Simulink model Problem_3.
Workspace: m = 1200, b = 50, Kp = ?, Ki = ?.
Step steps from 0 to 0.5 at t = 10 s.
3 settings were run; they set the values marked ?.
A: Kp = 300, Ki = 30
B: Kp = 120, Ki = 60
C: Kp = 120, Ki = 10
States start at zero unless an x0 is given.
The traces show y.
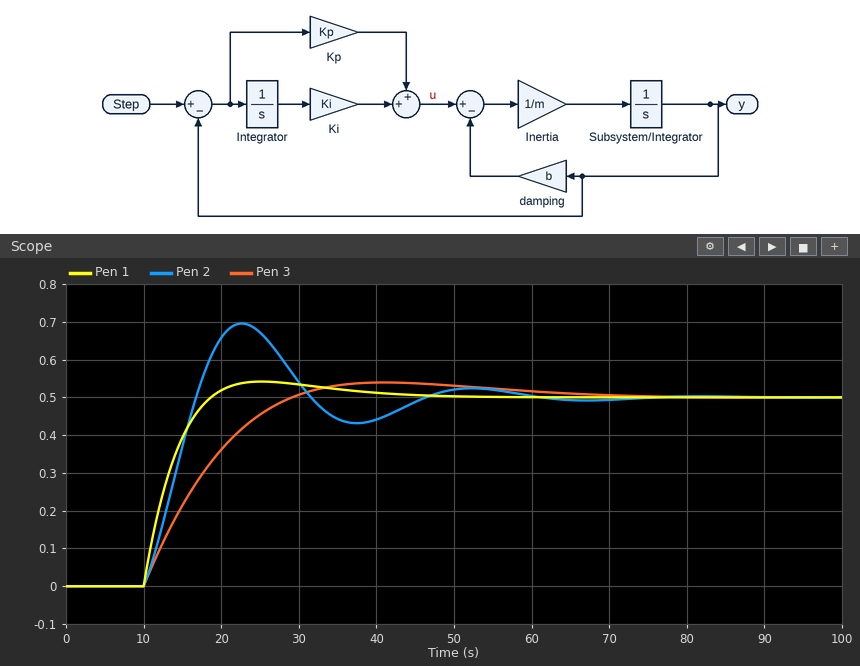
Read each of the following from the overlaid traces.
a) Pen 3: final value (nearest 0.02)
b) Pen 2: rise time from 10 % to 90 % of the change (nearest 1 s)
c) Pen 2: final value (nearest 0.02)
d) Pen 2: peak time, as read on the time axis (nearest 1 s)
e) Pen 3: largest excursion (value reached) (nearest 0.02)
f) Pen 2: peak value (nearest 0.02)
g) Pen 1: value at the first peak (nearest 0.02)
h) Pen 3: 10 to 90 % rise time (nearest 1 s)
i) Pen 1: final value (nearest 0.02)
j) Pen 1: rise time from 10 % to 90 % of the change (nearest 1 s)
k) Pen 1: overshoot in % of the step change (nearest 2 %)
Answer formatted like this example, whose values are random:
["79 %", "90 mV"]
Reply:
["0.50", "5 s", "0.50", "23 s", "0.54", "0.70", "0.54", "14 s", "0.50", "6 s", "8 %"]
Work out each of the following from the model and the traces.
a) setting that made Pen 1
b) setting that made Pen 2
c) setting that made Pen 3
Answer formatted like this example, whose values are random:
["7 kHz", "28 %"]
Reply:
["A", "B", "C"]
